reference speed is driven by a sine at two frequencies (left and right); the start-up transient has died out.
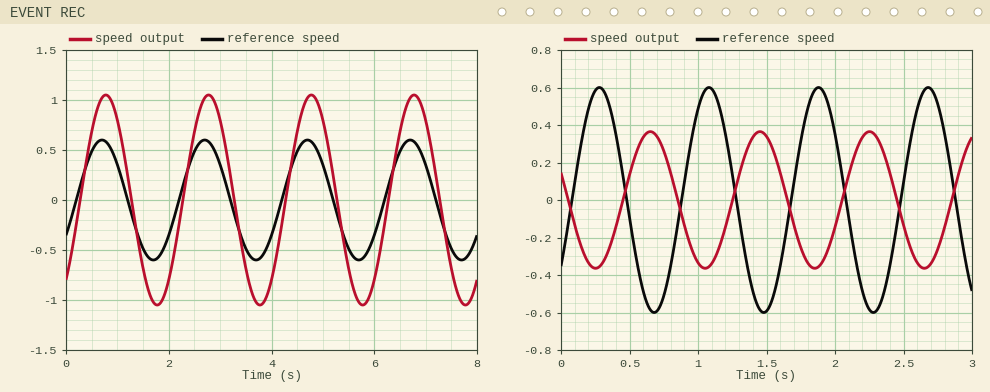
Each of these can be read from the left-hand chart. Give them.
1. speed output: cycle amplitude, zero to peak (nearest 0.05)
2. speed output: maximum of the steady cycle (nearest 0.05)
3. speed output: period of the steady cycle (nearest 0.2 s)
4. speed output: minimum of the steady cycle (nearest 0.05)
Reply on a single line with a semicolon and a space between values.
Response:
1.05; 1.05; 2.0 s; -1.05
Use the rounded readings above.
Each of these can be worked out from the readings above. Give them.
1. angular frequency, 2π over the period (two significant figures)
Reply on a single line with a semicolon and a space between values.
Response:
3.1 rad/s
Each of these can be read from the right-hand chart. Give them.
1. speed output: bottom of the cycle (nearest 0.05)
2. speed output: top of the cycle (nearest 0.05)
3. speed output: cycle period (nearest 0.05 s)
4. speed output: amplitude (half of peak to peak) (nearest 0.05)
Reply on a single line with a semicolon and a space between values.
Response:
-0.35; 0.35; 0.80 s; 0.35
